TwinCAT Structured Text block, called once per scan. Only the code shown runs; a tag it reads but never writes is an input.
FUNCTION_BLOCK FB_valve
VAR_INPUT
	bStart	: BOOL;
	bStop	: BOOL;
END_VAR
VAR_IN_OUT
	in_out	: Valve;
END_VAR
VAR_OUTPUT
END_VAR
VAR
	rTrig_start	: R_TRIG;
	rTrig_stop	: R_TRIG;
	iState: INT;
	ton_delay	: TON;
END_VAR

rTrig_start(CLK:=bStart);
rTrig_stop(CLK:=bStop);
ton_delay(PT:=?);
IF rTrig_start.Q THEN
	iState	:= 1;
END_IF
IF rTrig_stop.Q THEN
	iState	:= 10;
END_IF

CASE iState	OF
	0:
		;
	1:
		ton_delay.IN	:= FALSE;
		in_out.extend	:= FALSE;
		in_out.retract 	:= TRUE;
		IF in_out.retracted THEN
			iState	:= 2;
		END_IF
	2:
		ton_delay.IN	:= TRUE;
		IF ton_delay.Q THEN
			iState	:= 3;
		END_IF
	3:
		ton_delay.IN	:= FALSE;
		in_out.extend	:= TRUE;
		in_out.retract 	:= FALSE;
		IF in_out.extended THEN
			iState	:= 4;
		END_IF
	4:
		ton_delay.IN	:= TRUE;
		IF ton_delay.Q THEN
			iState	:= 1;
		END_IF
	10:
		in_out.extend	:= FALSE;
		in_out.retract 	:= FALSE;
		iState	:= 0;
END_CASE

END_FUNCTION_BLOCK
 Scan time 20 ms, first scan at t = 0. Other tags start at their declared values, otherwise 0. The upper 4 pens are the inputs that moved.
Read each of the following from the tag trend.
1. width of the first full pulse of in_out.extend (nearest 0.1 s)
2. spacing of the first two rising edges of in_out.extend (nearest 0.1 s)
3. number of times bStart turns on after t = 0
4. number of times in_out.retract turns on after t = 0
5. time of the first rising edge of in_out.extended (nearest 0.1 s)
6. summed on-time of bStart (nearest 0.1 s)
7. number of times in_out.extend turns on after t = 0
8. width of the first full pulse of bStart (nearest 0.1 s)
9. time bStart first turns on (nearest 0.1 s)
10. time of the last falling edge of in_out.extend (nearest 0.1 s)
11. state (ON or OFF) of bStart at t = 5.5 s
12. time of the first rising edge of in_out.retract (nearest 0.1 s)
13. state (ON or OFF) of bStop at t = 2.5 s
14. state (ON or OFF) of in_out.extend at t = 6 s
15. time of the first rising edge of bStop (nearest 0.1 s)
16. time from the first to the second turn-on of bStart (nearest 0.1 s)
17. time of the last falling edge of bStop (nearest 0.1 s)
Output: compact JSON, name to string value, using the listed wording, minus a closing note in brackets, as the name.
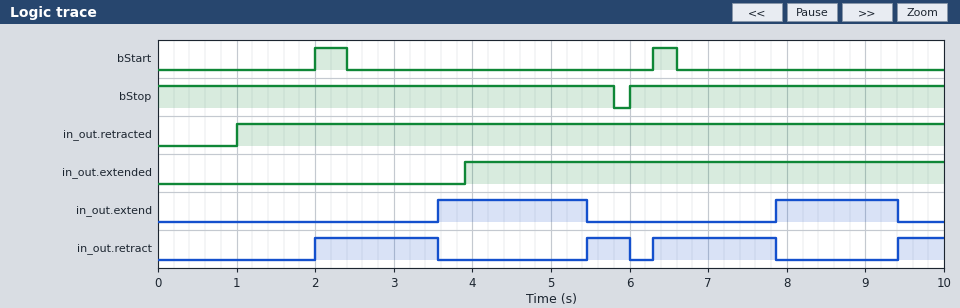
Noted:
{"width of the first full pulse of in_out.extend": "1.9 s", "spacing of the first two rising edges of in_out.extend": "4.3 s", "number of times bStart turns on after t = 0": "2", "number of times in_out.retract turns on after t = 0": "4", "time of the first rising edge of in_out.extended": "3.9 s", "summed on-time of bStart": "0.7 s", "number of times in_out.extend turns on after t = 0": "2", "width of the first full pulse of bStart": "0.4 s", "time bStart first turns on": "2.0 s", "time of the last falling edge of in_out.extend": "9.4 s", "state (ON or OFF) of bStart at t = 5.5 s": "OFF", "time of the first rising edge of in_out.retract": "2.0 s", "state (ON or OFF) of bStop at t = 2.5 s": "ON", "state (ON or OFF) of in_out.extend at t = 6 s": "OFF", "time of the first rising edge of bStop": "6.0 s", "time from the first to the second turn-on of bStart": "4.3 s", "time of the last falling edge of bStop": "5.8 s"}
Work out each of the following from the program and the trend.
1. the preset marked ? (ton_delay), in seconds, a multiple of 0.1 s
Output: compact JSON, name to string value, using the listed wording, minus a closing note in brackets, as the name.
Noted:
{"the preset marked ? (ton_delay), in seconds, a multiple of 0.1 s": "1.5 s"}
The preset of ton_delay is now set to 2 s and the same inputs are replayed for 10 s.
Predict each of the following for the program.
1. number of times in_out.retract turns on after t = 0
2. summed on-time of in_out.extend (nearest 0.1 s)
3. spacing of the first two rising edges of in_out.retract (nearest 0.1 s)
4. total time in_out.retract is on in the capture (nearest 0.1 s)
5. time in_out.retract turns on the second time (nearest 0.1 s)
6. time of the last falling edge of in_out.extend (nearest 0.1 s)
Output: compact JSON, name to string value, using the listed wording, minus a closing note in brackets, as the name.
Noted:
{"number of times in_out.retract turns on after t = 0": "2", "summed on-time of in_out.extend": "3.6 s", "spacing of the first two rising edges of in_out.retract": "4.3 s", "total time in_out.retract is on in the capture": "4.1 s", "time in_out.retract turns on the second time": "6.3 s", "time of the last falling edge of in_out.extend": "6.0 s"}
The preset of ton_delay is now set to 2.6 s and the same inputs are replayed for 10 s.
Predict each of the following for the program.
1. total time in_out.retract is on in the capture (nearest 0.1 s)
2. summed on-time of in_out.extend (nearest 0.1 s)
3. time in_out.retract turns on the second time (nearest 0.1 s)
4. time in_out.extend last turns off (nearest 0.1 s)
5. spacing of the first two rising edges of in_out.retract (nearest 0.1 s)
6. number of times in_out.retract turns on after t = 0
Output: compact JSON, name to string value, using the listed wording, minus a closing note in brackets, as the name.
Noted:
{"total time in_out.retract is on in the capture": "5.3 s", "summed on-time of in_out.extend": "2.4 s", "time in_out.retract turns on the second time": "6.3 s", "time in_out.extend last turns off": "6.0 s", "spacing of the first two rising edges of in_out.retract": "4.3 s", "number of times in_out.retract turns on after t = 0": "2"}
